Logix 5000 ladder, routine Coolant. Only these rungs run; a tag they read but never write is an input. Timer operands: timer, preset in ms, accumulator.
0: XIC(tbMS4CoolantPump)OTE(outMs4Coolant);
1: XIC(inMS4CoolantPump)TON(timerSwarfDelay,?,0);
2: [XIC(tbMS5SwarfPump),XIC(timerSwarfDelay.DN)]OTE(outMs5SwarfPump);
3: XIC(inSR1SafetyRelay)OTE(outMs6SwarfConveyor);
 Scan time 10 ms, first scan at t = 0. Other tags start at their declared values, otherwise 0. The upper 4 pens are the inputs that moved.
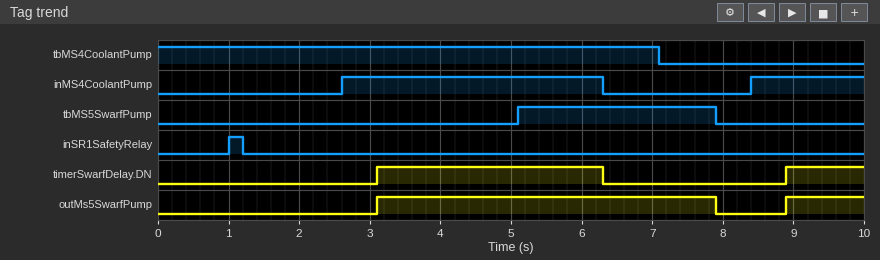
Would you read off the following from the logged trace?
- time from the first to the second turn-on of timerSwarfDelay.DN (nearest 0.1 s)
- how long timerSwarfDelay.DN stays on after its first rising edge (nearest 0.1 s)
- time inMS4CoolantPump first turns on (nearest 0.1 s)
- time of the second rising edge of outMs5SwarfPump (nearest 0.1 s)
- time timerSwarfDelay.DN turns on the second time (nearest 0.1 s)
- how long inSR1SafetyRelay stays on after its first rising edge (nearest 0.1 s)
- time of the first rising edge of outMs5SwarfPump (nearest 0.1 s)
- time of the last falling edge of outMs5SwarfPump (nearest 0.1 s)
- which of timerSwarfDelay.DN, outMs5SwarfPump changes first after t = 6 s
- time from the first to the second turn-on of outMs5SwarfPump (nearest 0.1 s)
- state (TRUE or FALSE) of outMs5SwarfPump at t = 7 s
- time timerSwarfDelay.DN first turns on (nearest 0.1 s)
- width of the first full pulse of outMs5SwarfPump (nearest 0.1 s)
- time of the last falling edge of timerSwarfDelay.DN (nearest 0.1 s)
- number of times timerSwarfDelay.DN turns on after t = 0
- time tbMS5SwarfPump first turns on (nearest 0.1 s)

5.8 s
3.2 s
2.6 s
8.9 s
8.9 s
0.2 s
3.1 s
7.9 s
timerSwarfDelay.DN
5.8 s
TRUE
3.1 s
4.8 s
6.3 s
2
5.1 s
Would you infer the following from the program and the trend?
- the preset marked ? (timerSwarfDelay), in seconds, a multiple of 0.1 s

0.5 s
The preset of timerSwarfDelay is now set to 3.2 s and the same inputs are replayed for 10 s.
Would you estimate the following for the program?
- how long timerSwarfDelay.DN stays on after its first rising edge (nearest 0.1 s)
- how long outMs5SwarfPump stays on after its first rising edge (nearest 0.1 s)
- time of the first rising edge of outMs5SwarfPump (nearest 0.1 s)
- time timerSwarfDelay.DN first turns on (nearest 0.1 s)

0.5 s
2.8 s
5.1 s
5.8 s
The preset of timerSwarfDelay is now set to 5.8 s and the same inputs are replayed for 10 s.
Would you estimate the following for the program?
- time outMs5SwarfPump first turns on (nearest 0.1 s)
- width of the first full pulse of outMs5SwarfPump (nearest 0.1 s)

5.1 s
2.8 s
